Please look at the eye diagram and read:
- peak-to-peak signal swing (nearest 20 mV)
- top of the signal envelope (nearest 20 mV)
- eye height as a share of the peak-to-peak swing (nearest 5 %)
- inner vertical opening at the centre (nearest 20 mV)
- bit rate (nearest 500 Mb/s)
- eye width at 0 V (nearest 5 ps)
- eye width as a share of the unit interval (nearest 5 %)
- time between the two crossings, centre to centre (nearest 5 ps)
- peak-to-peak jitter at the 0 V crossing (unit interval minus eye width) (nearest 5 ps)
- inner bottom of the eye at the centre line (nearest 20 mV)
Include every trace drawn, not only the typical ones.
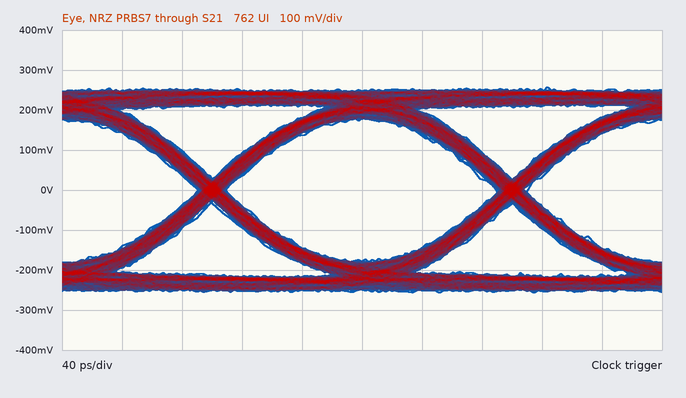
520 mV
260 mV
70 %
360 mV
5.0 Gb/s
180 ps
90 %
200 ps
20 ps
-180 mV
